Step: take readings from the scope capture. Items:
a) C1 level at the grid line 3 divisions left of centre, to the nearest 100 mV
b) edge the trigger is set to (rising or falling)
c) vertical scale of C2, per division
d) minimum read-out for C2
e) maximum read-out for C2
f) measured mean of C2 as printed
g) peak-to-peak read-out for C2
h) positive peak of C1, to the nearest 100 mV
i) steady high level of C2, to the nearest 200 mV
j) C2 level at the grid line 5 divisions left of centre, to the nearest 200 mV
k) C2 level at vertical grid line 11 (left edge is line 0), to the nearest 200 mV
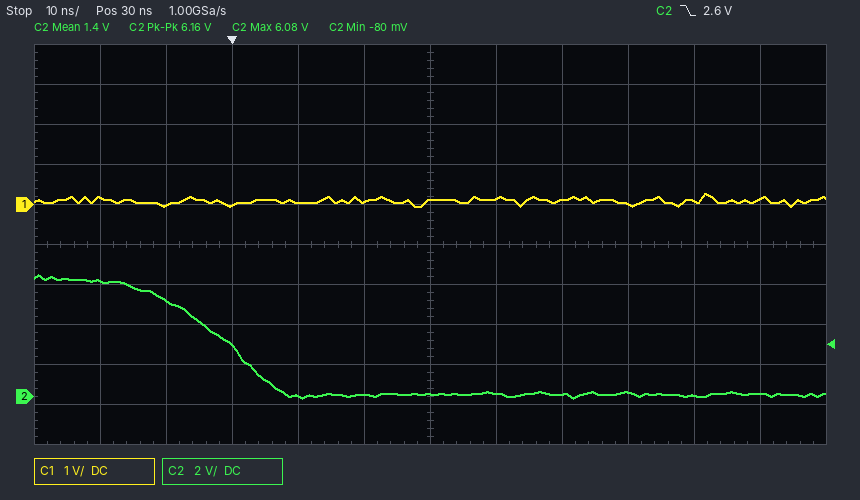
0.0 V
falling
2 V
-80 mV
6.08 V
1.4 V
6.16 V
300 mV
5.8 V
5.8 V
200 mV
